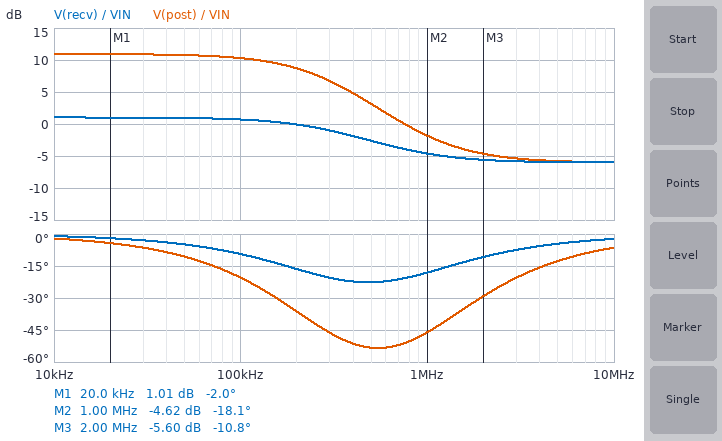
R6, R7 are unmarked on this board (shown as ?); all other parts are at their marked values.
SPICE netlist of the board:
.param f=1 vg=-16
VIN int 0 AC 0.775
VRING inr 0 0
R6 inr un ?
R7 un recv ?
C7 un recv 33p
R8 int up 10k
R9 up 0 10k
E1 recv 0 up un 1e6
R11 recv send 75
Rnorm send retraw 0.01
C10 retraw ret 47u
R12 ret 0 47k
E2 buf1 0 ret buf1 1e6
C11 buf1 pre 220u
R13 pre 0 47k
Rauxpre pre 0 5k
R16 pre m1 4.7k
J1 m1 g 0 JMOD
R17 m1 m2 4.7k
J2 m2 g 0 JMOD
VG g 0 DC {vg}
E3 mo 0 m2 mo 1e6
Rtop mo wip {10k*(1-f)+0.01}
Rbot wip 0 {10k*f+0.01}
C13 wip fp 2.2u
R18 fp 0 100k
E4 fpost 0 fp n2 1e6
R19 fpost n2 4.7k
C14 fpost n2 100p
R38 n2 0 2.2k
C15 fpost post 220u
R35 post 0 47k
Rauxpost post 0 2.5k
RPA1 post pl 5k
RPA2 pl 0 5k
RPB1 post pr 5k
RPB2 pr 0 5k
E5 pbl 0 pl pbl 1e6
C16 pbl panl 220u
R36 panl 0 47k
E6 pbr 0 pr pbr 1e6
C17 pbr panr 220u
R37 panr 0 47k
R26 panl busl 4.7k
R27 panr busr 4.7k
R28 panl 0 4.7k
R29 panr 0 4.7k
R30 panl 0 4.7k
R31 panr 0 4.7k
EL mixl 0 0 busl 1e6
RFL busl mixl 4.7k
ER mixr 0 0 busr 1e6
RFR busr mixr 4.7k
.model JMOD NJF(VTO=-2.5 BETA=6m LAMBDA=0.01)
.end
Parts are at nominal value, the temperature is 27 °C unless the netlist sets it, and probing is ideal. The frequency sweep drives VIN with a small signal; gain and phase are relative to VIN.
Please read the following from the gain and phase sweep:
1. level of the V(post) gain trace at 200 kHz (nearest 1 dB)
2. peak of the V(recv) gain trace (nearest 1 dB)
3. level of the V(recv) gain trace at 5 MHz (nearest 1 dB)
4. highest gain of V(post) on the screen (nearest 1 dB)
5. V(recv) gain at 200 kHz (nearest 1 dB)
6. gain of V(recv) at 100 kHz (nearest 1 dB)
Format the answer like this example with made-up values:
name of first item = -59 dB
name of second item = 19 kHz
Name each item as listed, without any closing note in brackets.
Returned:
level of the V(post) gain trace at 200 kHz = 9 dB
peak of the V(recv) gain trace = 1 dB
level of the V(recv) gain trace at 5 MHz = -6 dB
highest gain of V(post) on the screen = 11 dB
V(recv) gain at 200 kHz = 0 dB
gain of V(recv) at 100 kHz = 1 dB
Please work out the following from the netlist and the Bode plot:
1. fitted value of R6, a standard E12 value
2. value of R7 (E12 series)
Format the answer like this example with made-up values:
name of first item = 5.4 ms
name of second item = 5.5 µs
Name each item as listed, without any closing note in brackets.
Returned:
fitted value of R6, a standard E12 value = 12 kΩ
value of R7 = 15 kΩ
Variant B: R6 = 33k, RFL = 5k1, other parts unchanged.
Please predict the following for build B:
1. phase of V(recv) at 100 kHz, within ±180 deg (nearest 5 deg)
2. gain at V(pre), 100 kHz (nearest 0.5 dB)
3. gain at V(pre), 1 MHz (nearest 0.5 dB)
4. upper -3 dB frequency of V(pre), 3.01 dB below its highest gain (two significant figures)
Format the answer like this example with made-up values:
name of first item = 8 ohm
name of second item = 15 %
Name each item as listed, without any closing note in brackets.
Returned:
phase of V(recv) at 100 kHz, within ±180 deg = -5 deg
gain at V(pre), 100 kHz = -3.0 dB
gain at V(pre), 1 MHz = -5.5 dB
upper -3 dB frequency of V(pre), 3.01 dB below its highest gain = 1.4 MHz
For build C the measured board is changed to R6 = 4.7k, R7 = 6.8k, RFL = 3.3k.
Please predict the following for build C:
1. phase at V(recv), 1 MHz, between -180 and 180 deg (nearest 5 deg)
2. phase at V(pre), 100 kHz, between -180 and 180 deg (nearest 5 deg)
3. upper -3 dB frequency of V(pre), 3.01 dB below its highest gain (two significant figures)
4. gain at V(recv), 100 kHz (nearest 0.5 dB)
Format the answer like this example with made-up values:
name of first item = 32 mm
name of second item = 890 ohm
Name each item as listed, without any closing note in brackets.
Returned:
phase at V(recv), 1 MHz, between -180 and 180 deg = -25 deg
phase at V(pre), 100 kHz, between -180 and 180 deg = -5 deg
upper -3 dB frequency of V(pre), 3.01 dB below its highest gain = 870 kHz
gain at V(recv), 100 kHz = 1.5 dB
